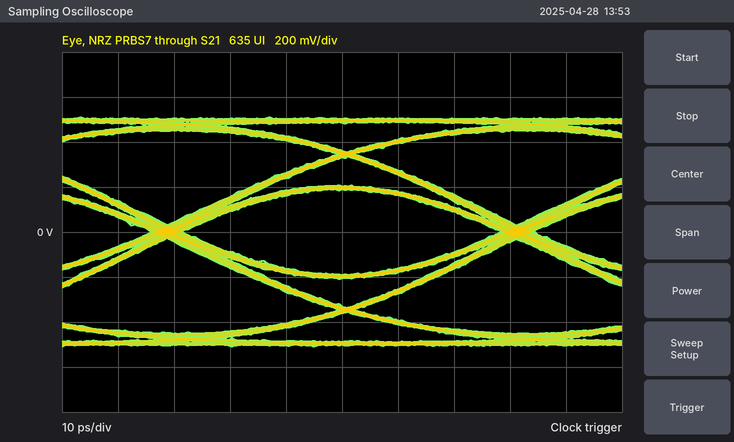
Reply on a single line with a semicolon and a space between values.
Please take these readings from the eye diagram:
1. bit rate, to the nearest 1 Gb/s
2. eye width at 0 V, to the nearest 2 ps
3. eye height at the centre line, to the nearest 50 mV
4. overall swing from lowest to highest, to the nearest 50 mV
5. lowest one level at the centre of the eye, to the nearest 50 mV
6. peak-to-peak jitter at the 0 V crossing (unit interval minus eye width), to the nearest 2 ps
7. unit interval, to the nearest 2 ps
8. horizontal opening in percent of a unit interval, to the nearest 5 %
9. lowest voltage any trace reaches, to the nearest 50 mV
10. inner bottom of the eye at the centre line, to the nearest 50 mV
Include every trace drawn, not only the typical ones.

16 Gb/s; 56 ps; 400 mV; 1.00 V; 200 mV; 6 ps; 62 ps; 90 %; -500 mV; -200 mV
